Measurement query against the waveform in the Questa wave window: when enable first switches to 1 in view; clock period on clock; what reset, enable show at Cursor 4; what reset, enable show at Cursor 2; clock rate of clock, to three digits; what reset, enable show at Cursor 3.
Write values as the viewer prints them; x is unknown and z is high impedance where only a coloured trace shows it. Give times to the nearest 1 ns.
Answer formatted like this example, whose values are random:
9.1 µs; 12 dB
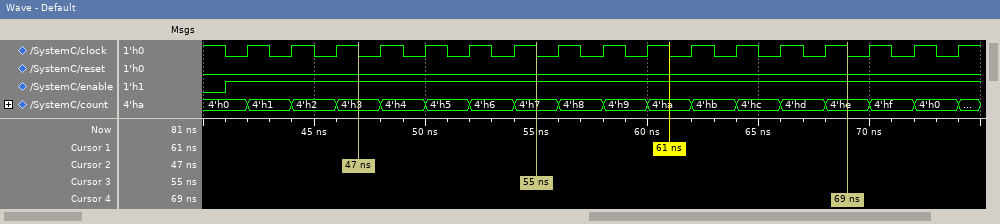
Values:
41 ns; 2 ns; reset=0, enable=1; reset=0, enable=1; 500 MHz; reset=0, enable=1
